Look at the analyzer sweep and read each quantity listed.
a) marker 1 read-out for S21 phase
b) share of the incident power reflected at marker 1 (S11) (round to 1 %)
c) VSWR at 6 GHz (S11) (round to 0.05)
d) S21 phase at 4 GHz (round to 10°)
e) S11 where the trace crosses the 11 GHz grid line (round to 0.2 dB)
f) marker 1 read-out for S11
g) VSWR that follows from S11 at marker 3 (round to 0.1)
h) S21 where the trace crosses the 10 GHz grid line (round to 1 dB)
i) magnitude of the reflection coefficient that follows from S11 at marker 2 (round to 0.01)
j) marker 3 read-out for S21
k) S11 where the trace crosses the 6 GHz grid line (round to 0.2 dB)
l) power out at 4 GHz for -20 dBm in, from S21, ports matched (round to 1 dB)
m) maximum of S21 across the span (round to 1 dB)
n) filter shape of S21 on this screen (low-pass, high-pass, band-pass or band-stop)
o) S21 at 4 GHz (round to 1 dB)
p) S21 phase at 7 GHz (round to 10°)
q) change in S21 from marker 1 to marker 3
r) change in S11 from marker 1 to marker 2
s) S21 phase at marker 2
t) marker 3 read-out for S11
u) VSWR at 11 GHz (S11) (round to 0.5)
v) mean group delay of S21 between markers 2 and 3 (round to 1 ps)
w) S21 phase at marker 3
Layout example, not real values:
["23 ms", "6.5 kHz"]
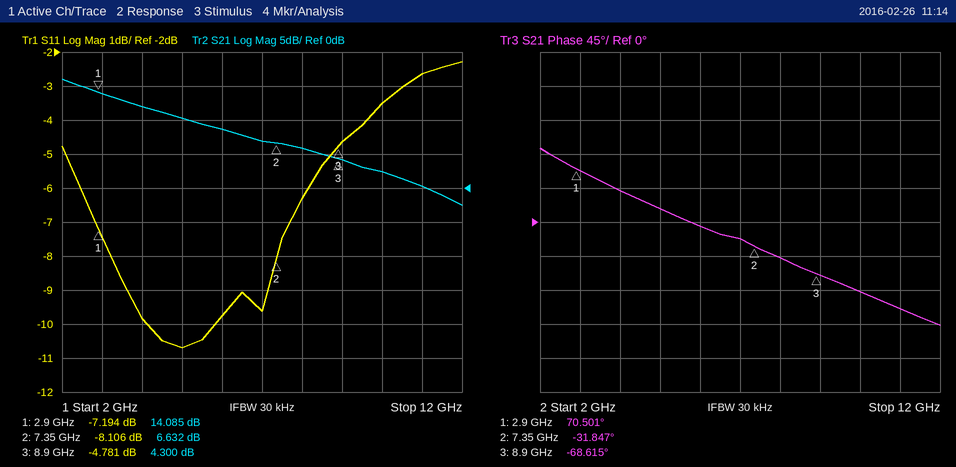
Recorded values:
["70.501°", "19 %", "1.95", "40°", "-2.6 dB", "-7.194 dB", "3.7", "2 dB", "0.39", "4.300 dB", "-9.8 dB", "-8 dBm", "16 dB", "low-pass", "12 dB", "-20°", "-9.785 dB", "-0.912 dB", "-31.847°", "-4.781 dB", "6.5", "66 ps", "-68.615°"]
